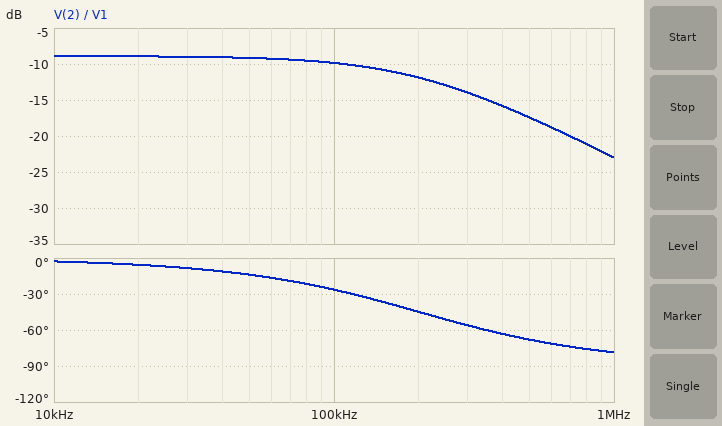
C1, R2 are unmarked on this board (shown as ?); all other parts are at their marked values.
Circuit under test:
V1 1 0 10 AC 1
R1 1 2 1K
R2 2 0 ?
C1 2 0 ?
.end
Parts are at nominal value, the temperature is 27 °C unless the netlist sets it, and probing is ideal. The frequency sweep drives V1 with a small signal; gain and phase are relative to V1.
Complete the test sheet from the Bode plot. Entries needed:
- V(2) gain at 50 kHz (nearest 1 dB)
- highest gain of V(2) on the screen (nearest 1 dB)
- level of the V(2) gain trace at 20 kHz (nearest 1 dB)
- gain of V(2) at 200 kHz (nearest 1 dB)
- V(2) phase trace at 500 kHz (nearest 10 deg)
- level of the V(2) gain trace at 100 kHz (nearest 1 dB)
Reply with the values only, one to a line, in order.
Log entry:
-9 dB
-9 dB
-9 dB
-12 dB
-70 deg
-10 dB
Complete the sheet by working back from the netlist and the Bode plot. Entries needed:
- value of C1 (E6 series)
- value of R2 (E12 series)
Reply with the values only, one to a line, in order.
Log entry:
2.2 nF
560 Ω
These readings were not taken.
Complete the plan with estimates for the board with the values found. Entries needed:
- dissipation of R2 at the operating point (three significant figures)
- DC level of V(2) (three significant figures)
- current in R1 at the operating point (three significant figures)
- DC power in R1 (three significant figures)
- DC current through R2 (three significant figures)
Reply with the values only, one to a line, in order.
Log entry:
23.0 mW
3.59 V
6.41 mA
41.1 mW
6.41 mA
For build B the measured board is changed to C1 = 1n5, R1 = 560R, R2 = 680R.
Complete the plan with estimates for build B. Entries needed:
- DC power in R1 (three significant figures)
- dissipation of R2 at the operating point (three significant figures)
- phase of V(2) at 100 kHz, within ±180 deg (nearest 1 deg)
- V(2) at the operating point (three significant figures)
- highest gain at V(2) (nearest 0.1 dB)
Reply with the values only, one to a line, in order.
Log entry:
36.4 mW
44.2 mW
-16 deg
5.48 V
-5.2 dB
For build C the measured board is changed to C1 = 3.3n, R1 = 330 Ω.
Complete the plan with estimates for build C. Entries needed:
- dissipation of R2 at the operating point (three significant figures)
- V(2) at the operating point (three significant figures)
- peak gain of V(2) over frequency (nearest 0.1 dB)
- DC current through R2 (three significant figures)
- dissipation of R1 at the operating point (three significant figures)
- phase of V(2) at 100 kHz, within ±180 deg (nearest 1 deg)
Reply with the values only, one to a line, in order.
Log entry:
70.7 mW
6.29 V
-4.0 dB
11.2 mA
41.7 mW
-23 deg
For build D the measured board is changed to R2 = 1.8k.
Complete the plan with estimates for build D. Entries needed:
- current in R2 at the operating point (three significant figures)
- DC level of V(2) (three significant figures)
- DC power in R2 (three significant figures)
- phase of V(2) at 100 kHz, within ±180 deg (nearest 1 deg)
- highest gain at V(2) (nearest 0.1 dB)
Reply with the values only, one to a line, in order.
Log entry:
3.57 mA
6.43 V
23.0 mW
-42 deg
-3.8 dB
